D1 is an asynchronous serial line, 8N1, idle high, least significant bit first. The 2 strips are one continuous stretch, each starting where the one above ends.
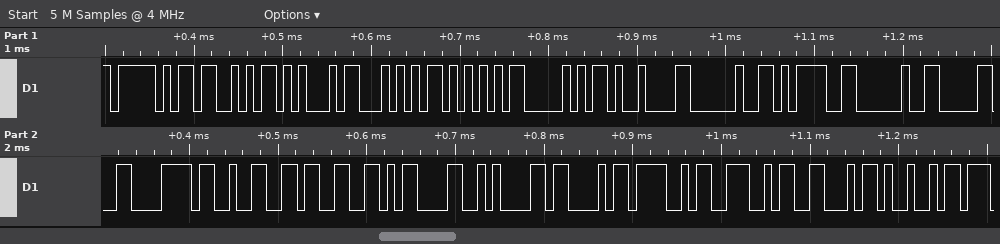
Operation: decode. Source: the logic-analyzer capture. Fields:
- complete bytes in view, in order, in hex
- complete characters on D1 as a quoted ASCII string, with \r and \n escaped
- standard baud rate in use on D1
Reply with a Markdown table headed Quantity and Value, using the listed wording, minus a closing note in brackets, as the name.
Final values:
| Quantity | Value |
|---|---|
| complete bytes in view, in order, in hex | 5F 53 45 54 55 50 09 20 3D 20 30 78 32 33 0D 0A 43 4F 4E 46 49 |
| complete characters on D1 as a quoted ASCII string, with \r and \n escaped | "_SETUP\t = 0x23\r\nCONFI" |
| standard baud rate in use on D1 | 115200 baud |
